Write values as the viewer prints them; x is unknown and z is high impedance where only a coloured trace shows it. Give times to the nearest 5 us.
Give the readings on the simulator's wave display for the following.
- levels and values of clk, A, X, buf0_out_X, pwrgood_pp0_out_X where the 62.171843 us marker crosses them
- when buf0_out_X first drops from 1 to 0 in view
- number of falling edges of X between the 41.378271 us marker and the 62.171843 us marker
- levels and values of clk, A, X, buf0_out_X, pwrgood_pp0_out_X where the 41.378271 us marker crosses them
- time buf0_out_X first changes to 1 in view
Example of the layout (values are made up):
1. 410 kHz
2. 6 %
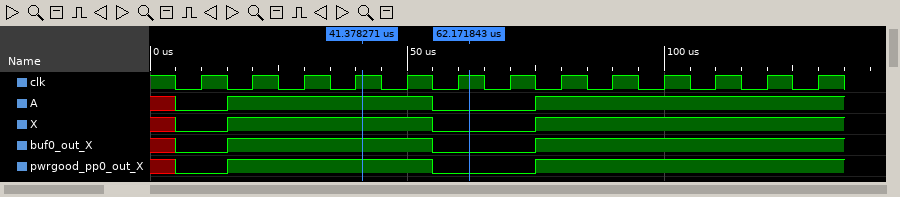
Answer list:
1. clk=1, A=0, X=0, buf0_out_X=0, pwrgood_pp0_out_X=0
2. 55 us
3. 1
4. clk=1, A=1, X=1, buf0_out_X=1, pwrgood_pp0_out_X=1
5. 15 us
